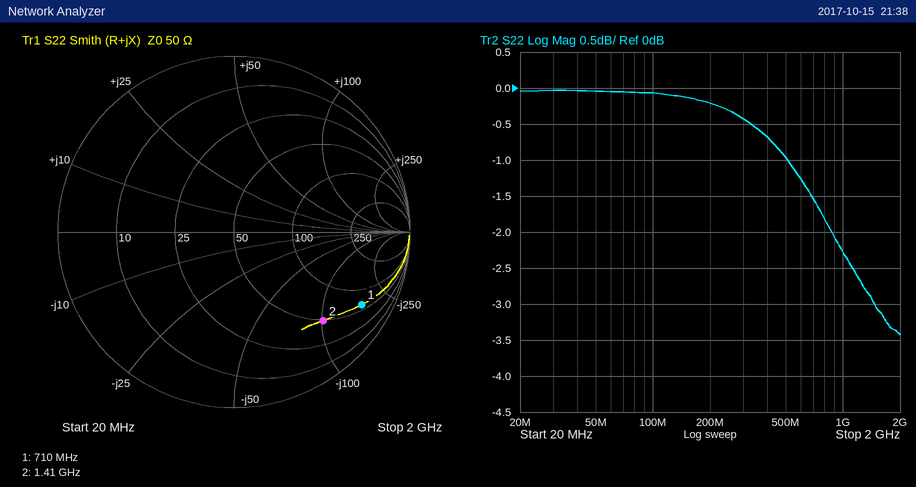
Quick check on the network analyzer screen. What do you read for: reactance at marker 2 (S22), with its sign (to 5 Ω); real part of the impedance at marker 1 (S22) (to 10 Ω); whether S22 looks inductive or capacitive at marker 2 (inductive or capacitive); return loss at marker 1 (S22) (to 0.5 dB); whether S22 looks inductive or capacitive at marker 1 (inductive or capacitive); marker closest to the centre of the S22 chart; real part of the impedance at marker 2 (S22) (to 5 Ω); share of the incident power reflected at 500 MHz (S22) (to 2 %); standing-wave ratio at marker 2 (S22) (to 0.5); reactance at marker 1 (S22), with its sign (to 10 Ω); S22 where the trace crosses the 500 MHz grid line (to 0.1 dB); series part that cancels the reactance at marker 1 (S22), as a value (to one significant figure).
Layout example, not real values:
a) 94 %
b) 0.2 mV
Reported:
a) -100 Ω
b) 60 Ω
c) capacitive
d) 1.5 dB
e) capacitive
f) marker 2
g) 50 Ω
h) 80 %
i) 6.0
j) -170 Ω
k) -1.0 dB
l) 40 nH
